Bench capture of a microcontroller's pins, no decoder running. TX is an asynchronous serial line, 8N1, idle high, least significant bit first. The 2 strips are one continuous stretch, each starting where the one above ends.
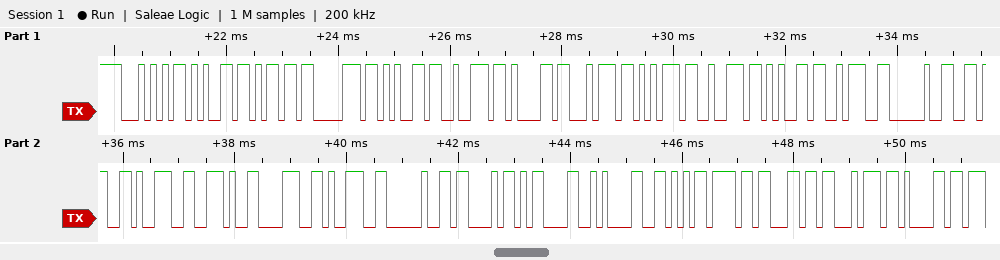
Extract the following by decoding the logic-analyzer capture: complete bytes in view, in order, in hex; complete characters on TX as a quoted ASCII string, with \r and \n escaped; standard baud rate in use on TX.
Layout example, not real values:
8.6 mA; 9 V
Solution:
54 65 6D 70 65 72 61 74 75 72 65 3A 20 36 39 2E 38 39 20 43 0D 0A 56 6F 6C 74 61; "Temperature: 69.89 C\r\nVolta"; 9600 baud
